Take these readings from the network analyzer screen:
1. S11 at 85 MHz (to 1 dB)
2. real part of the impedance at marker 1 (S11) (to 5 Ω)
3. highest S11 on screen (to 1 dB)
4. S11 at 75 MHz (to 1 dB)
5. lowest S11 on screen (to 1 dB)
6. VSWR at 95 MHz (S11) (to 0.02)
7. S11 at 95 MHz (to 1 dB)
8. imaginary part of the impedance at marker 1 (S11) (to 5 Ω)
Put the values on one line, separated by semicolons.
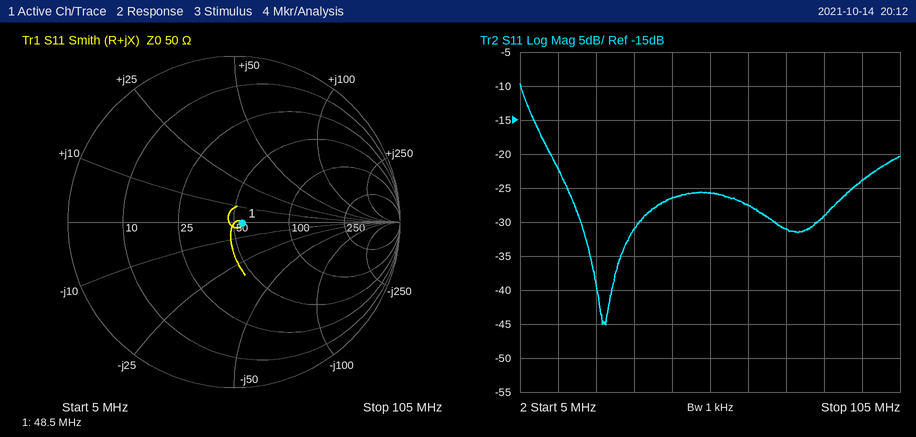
-29 dB; 55 Ω; -10 dB; -31 dB; -45 dB; 1.14; -24 dB; 0 Ω
